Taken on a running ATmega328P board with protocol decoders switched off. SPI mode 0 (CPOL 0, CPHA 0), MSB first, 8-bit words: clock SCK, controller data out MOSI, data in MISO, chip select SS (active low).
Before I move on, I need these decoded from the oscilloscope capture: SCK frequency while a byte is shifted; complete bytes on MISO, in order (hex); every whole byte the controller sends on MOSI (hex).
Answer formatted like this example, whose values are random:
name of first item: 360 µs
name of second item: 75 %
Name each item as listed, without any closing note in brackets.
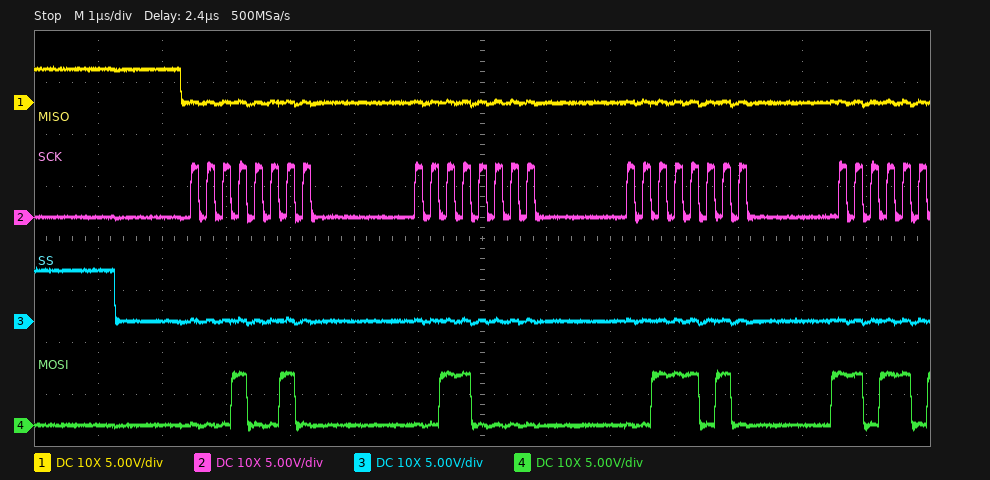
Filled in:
SCK frequency while a byte is shifted: 4 MHz
complete bytes on MISO, in order: 00 00 00
every whole byte the controller sends on MOSI: 12 30 3A
